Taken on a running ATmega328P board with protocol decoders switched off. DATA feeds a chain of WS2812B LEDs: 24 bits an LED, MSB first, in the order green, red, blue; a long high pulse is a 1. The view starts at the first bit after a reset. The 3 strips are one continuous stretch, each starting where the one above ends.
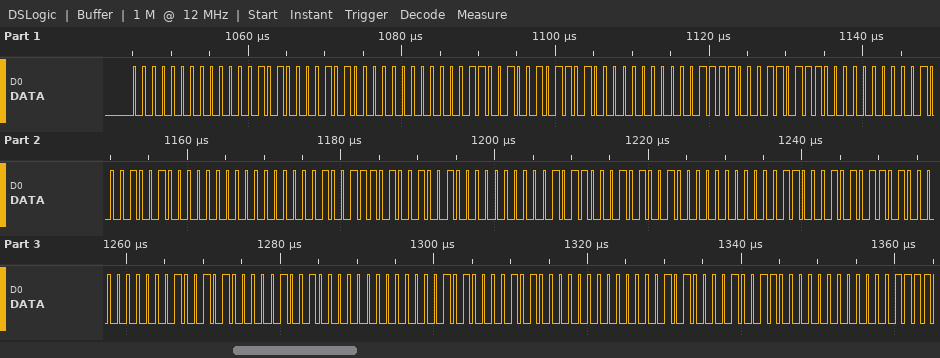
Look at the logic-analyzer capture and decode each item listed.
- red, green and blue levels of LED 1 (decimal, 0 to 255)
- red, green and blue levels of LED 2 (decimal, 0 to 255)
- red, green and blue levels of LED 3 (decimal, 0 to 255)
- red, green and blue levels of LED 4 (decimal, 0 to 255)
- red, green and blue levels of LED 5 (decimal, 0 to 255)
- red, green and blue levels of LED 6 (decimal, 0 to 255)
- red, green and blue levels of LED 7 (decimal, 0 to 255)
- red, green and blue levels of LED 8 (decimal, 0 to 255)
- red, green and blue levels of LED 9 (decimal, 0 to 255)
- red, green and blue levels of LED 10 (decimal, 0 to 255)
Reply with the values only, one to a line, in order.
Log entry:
5, 0, 10
25, 0, 45
30, 0, 55
34, 0, 64
39, 0, 73
44, 0, 82
49, 0, 90
74, 0, 9
5, 0, 10
10, 0, 19
